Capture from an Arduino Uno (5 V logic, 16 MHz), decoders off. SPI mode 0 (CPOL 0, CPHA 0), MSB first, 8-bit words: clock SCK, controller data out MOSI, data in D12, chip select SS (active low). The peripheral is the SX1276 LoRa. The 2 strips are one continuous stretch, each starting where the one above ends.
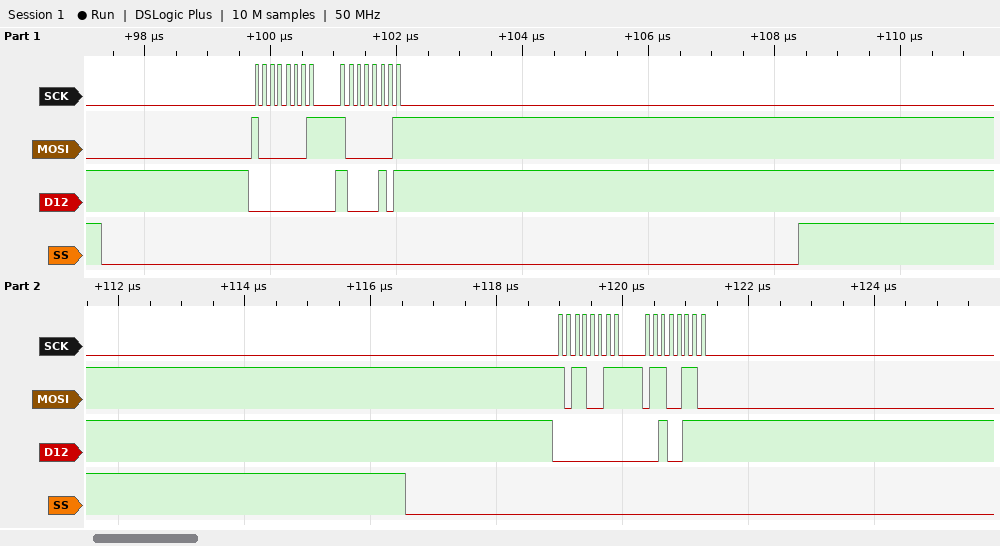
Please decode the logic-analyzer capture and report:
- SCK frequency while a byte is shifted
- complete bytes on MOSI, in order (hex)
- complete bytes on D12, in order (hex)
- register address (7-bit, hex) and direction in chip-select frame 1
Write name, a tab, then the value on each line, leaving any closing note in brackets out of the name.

SCK frequency while a byte is shifted	8 MHz
complete bytes on MOSI, in order	81 81 B3 66
complete bytes on D12, in order	00 85 00 27
register address (7-bit, hex) and direction in chip-select frame 1	0x01 write
